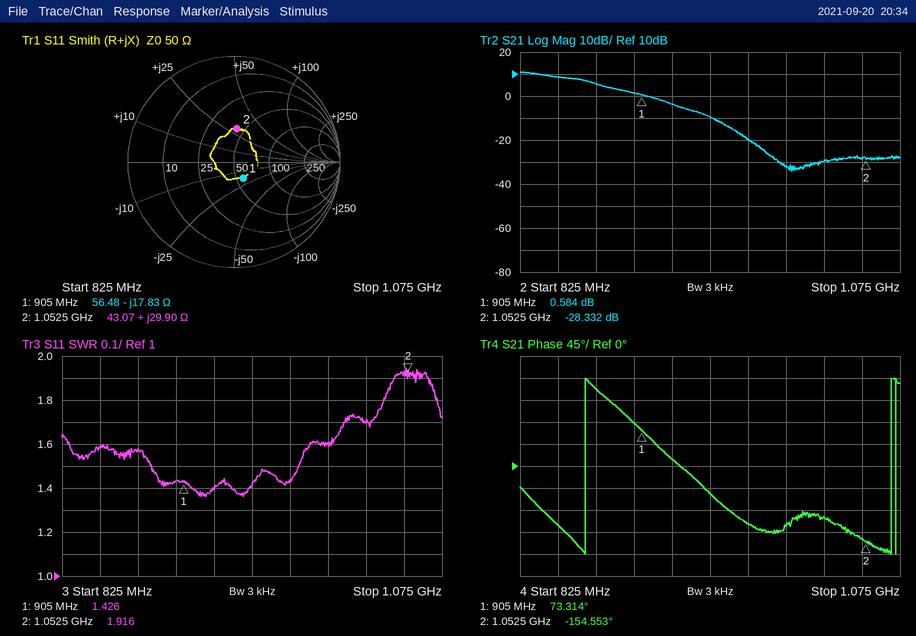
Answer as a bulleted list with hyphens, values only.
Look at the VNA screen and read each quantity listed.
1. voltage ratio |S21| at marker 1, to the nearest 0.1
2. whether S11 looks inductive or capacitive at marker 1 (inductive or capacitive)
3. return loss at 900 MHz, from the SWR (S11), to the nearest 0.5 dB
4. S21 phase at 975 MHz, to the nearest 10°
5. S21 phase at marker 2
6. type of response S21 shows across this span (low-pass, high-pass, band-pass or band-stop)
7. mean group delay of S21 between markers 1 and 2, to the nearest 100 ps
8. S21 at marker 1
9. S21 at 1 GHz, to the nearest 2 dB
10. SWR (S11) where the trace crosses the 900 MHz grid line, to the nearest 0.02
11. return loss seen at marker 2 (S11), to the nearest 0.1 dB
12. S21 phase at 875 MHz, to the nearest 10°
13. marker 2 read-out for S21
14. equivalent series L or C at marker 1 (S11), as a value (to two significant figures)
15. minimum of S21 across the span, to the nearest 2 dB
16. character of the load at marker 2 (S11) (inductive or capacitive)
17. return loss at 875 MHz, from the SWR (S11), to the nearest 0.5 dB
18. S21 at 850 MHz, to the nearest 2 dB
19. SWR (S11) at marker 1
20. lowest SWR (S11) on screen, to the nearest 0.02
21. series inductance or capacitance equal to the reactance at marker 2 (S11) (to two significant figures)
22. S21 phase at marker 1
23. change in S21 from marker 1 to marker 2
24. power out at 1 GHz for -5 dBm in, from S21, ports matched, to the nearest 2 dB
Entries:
- 1.1
- capacitive
- 15.0 dB
- -120°
- -154.553°
- low-pass
- 4.3 ns
- 0.584 dB
- -32 dB
- 1.44
- 10.1 dB
- 160°
- -28.332 dB
- 9.9 pF
- -34 dB
- inductive
- 13.0 dB
- 8 dB
- 1.426
- 1.36
- 4.5 nH
- 73.314°
- -28.916 dB
- -36 dBm
